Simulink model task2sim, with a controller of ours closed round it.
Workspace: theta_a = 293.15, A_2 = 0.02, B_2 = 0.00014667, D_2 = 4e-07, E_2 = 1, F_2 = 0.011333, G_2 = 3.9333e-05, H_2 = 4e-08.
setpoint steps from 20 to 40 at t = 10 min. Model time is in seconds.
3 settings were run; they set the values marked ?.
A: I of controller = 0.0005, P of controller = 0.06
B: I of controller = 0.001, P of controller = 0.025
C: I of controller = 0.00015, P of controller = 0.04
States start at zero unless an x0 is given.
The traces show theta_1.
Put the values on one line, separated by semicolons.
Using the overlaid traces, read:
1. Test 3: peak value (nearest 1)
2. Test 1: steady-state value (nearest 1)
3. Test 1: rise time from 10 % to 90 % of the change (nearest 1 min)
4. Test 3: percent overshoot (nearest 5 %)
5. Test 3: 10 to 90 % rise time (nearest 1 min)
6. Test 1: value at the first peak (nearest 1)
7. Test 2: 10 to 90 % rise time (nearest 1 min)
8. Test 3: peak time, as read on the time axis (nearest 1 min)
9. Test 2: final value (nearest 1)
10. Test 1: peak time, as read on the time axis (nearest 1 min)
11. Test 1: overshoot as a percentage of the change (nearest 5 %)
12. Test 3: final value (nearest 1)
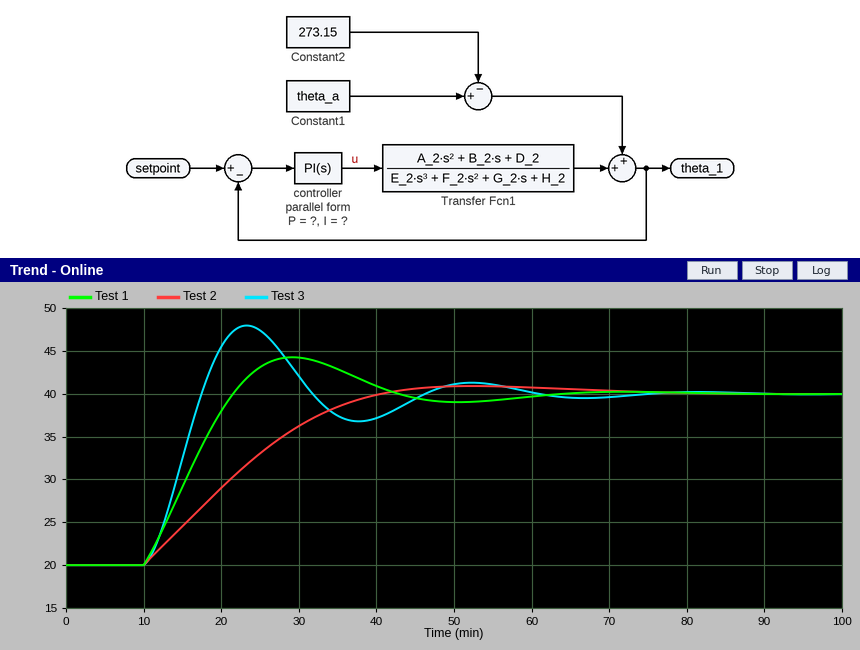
48; 40; 9 min; 40 %; 5 min; 44; 22 min; 23 min; 40; 29 min; 20 %; 40
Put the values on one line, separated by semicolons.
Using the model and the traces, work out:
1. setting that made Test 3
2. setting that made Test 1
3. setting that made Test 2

B; A; C
